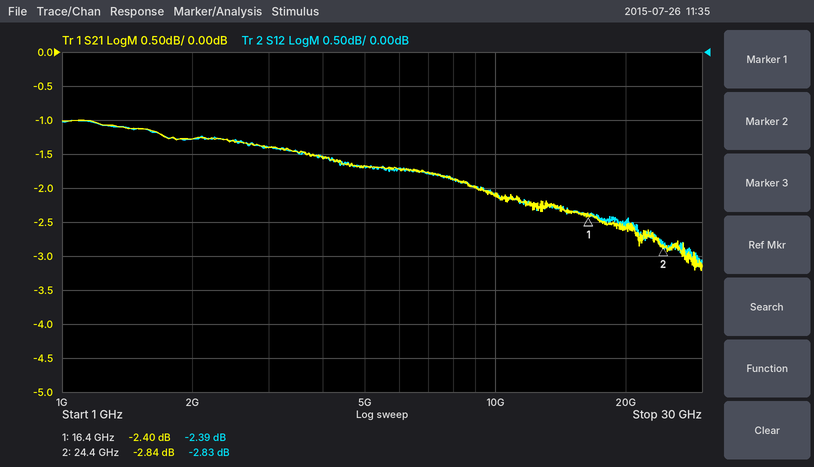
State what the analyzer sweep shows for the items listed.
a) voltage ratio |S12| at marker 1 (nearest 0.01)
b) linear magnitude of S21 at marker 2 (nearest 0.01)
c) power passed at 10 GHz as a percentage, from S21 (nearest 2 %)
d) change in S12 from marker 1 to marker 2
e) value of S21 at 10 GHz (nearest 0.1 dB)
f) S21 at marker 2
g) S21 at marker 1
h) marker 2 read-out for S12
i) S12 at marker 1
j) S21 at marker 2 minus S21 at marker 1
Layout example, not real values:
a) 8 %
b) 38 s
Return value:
a) 0.76
b) 0.72
c) 62 %
d) -0.44 dB
e) -2.1 dB
f) -2.84 dB
g) -2.40 dB
h) -2.83 dB
i) -2.39 dB
j) -0.44 dB
